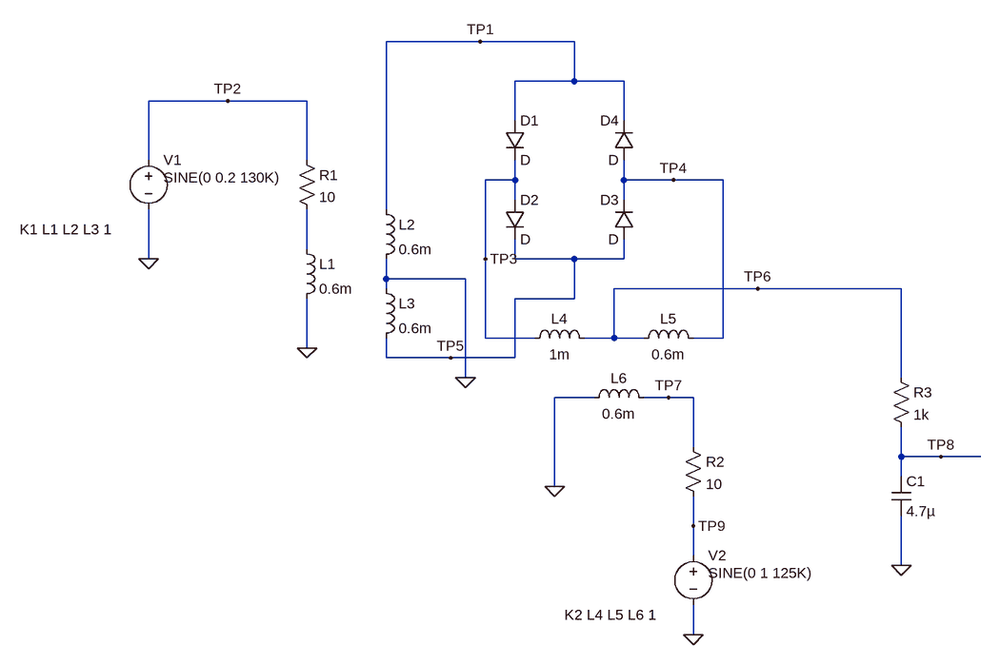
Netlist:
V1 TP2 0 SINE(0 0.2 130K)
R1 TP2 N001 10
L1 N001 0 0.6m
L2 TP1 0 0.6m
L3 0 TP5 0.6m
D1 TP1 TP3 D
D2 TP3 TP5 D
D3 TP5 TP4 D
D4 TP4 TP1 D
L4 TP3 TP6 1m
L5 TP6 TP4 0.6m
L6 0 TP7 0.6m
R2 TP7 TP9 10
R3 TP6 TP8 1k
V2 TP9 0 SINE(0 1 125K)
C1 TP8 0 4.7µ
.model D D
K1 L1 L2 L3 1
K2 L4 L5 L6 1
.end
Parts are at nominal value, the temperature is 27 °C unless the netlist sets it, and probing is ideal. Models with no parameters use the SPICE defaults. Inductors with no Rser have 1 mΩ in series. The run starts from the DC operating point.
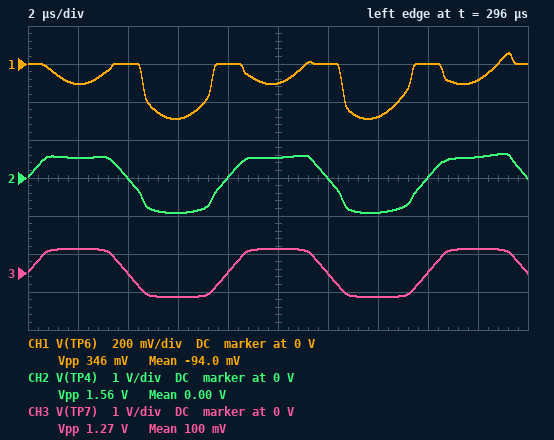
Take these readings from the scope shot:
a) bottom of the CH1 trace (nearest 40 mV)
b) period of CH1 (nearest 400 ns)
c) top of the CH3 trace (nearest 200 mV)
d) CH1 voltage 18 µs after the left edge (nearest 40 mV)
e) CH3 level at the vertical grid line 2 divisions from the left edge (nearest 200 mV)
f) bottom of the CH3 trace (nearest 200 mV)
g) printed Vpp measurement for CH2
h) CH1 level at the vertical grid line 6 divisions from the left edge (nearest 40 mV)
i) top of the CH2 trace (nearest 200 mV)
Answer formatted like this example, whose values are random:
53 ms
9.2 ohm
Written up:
-280 mV
8.0 µs
600 mV
-80 mV
0 V
-600 mV
1.56 V
0 V
600 mV
